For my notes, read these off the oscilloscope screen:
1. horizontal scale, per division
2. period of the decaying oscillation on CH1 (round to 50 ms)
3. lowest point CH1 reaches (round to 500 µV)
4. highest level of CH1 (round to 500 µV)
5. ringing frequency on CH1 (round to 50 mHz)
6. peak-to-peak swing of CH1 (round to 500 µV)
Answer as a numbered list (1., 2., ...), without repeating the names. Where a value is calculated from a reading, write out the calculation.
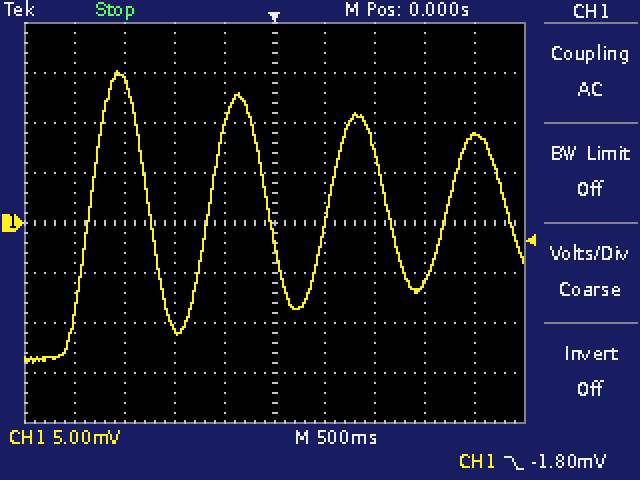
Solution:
1. 500 ms
2. 1.20 s
3. -14.0 mV
4. 15.0 mV
5. 1 / 1.20 s ≈ 833 mHz, so 850 mHz to the nearest 50 mHz
6. 15.0 mV − (-14.0 mV) = 29.0 mV
